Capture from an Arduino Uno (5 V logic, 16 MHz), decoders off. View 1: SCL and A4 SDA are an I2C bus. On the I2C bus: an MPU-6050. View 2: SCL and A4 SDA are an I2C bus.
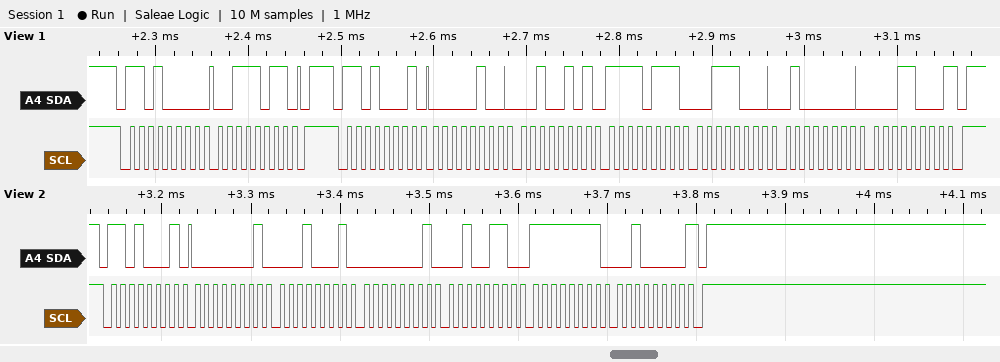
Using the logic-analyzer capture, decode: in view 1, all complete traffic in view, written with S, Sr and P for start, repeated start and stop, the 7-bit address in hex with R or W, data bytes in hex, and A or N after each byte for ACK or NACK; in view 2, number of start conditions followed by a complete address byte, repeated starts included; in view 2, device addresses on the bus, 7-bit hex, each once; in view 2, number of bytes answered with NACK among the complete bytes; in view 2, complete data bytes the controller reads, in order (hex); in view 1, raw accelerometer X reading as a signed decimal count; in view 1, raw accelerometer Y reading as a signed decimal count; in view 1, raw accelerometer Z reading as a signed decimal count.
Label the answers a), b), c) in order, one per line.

a) S 68W A 3B A P S 68R A 04 A 25 A F7 A 38 A 40 A 18 N P
b) 1
c) 0x68
d) 1
e) 01 11 01 26 FF 20
f) 1061
g) -2248
h) 16408
